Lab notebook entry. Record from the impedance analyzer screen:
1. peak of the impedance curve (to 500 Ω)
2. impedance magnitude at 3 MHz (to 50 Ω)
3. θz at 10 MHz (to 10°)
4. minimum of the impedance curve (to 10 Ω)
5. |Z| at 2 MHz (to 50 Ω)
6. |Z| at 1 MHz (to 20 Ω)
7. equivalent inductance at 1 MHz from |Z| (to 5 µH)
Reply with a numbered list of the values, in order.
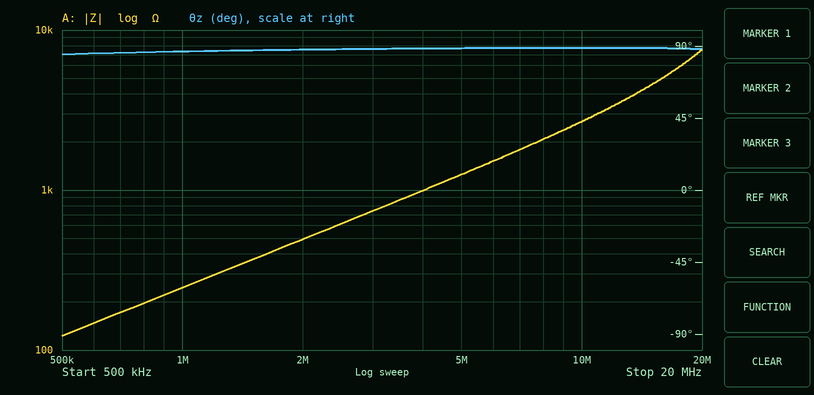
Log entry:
1. 7.5 kΩ
2. 750 Ω
3. 90°
4. 120 Ω
5. 500 Ω
6. 240 Ω
7. 40 µH
